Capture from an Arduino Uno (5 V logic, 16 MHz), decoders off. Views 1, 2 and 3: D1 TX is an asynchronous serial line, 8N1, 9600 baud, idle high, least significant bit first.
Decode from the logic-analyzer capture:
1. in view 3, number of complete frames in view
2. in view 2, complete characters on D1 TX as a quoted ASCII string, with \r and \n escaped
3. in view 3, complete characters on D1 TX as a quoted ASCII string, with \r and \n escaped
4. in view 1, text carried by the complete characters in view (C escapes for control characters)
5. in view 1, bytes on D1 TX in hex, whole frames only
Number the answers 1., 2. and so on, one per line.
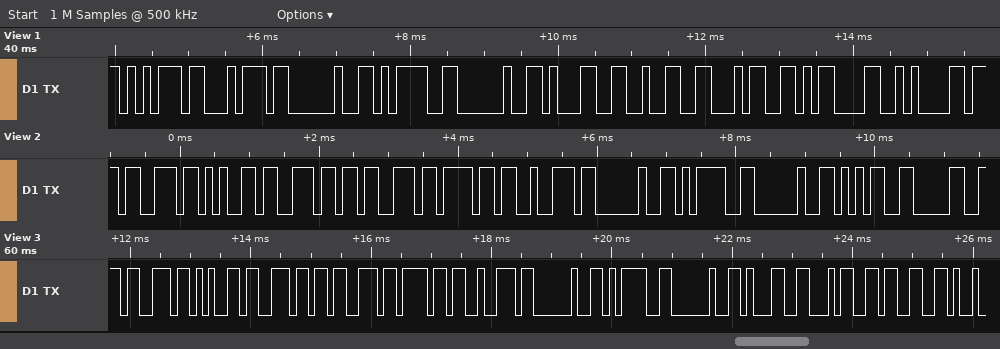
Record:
1. 12
2. "sensor = 50"
3. "sensor = 143"
4. "ut = 124\r\n"
5. 0x75 0x74 0x20 0x3D 0x20 0x31 0x32 0x34 0x0D 0x0A
